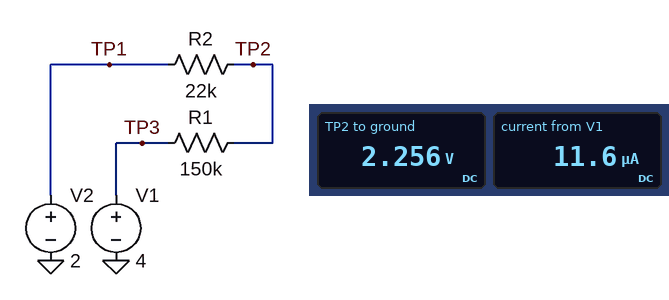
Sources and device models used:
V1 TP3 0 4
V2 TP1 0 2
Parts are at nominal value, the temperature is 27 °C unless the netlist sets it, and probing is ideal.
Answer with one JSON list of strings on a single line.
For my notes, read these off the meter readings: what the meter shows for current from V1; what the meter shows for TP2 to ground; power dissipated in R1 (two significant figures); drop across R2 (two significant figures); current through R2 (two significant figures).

["11.6 µA", "2.256 V", "20 µW", "260 mV", "12 µA"]
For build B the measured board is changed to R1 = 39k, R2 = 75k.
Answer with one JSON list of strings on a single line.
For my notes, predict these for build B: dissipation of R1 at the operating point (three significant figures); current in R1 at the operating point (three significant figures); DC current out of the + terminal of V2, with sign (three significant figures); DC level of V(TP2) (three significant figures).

["12.0 µW", "17.5 µA", "-17.5 µA", "3.32 V"]
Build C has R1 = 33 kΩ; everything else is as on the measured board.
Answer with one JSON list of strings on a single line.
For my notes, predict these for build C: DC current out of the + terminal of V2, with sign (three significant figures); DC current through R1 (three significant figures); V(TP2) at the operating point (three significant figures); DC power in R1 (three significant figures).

["-36.4 µA", "36.4 µA", "2.80 V", "43.6 µW"]
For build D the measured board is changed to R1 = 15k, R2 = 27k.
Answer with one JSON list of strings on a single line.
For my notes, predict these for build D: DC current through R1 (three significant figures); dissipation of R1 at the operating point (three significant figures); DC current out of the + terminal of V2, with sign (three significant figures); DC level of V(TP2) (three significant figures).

["47.6 µA", "34.0 µW", "-47.6 µA", "3.29 V"]
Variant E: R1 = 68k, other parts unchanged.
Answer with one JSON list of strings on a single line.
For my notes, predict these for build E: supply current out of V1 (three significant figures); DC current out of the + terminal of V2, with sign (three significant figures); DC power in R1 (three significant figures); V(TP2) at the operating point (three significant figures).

["22.2 µA", "-22.2 µA", "33.6 µW", "2.49 V"]
